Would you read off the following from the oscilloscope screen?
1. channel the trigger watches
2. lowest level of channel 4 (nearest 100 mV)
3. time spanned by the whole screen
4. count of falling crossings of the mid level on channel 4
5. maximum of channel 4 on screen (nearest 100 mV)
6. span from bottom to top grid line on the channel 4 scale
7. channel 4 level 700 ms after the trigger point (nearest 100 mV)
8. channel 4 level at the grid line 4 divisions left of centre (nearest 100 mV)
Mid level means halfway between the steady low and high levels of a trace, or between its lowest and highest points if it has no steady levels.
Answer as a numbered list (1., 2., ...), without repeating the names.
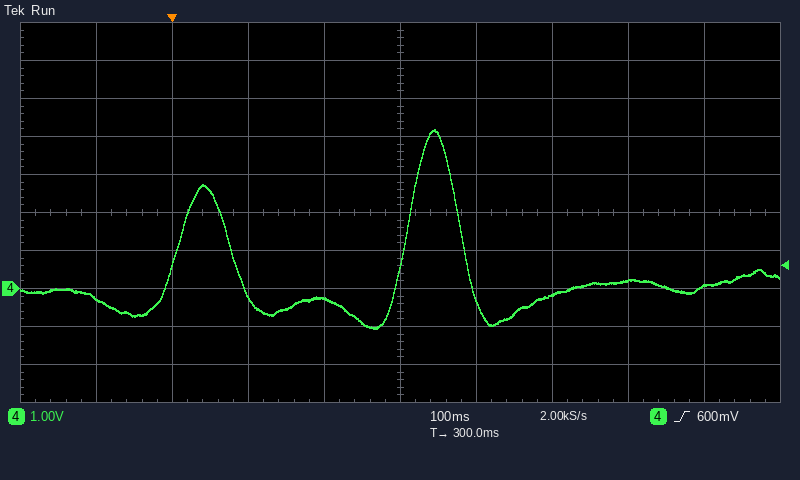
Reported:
1. channel 4
2. -1.1 V
3. 1 s
4. 2
5. 4.2 V
6. 10 V
7. 100 mV
8. -300 mV
